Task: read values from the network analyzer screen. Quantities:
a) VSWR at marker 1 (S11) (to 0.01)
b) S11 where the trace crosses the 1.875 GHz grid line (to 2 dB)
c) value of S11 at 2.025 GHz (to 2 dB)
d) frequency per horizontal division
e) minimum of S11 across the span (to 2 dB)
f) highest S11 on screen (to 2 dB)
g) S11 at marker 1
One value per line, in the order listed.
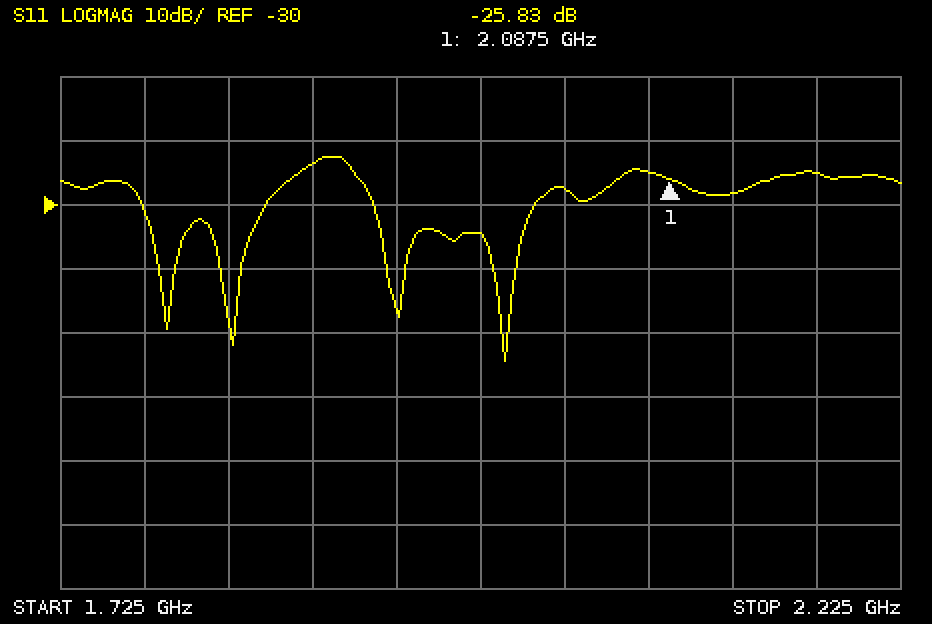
1.11
-24 dB
-28 dB
50 MHz
-54 dB
-22 dB
-25.83 dB
